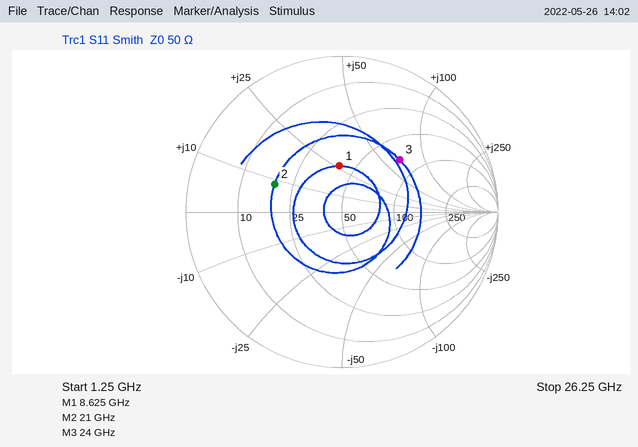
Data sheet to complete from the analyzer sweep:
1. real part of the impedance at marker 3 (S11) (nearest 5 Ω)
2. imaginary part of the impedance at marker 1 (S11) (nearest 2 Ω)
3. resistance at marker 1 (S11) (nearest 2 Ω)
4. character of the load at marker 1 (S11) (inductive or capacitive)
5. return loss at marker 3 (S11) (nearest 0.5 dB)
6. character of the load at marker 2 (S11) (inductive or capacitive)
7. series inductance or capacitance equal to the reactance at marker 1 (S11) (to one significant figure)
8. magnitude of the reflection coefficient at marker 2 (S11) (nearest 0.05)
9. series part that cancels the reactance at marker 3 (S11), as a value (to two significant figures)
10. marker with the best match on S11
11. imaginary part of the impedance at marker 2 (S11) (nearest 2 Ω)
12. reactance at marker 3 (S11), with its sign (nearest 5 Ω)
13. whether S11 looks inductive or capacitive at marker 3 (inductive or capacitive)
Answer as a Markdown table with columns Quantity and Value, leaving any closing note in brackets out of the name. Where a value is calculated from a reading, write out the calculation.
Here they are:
| Quantity | Value |
|---|---|
| real part of the impedance at marker 3 (S11) | 75 Ω |
| imaginary part of the impedance at marker 1 (S11) | +26 Ω |
| resistance at marker 1 (S11) | 40 Ω |
| character of the load at marker 1 (S11) | inductive |
| return loss at marker 3 (S11) | 6.0 dB |
| character of the load at marker 2 (S11) | inductive |
| series inductance or capacitance equal to the reactance at marker 1 (S11) | L = 26 Ω/(2π × 8.625 GHz) ≈ 480 pH, so 500 pH to one significant figure |
| magnitude of the reflection coefficient at marker 2 (S11) | 0.45 |
| series part that cancels the reactance at marker 3 (S11), as a value | C = 1/(2π × 24 GHz × 65 Ω) ≈ 102 fF, so 100 fF to two significant figures |
| marker with the best match on S11 | marker 1 |
| imaginary part of the impedance at marker 2 (S11) | +8 Ω |
| reactance at marker 3 (S11), with its sign | +65 Ω |
| whether S11 looks inductive or capacitive at marker 3 | inductive |
